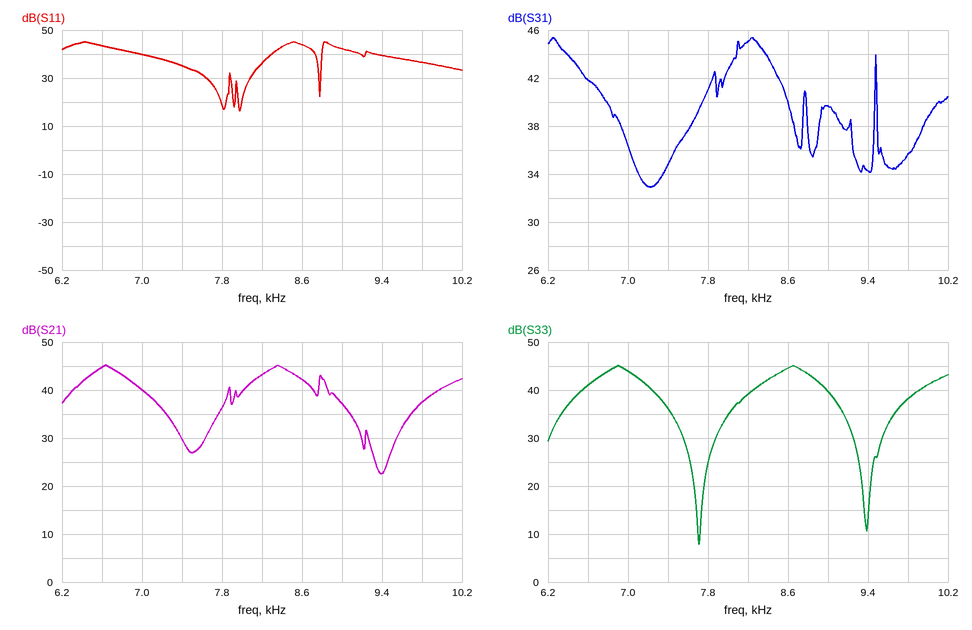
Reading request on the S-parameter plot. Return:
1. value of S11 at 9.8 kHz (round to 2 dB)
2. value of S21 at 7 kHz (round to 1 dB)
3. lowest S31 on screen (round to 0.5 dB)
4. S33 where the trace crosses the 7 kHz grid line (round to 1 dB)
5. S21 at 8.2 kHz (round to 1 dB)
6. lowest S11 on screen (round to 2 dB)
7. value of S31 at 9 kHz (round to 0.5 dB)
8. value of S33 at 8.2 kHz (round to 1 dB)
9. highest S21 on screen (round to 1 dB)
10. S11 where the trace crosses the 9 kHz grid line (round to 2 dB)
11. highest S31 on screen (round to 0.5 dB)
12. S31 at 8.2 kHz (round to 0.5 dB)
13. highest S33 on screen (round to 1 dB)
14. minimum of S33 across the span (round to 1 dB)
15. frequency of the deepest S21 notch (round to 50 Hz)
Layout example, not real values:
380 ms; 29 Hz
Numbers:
36 dB; 40 dB; 33.0 dB; 44 dB; 43 dB; 16 dB; 39.5 dB; 39 dB; 45 dB; 42 dB; 45.5 dB; 45.0 dB; 45 dB; 8 dB; 9.40 kHz
